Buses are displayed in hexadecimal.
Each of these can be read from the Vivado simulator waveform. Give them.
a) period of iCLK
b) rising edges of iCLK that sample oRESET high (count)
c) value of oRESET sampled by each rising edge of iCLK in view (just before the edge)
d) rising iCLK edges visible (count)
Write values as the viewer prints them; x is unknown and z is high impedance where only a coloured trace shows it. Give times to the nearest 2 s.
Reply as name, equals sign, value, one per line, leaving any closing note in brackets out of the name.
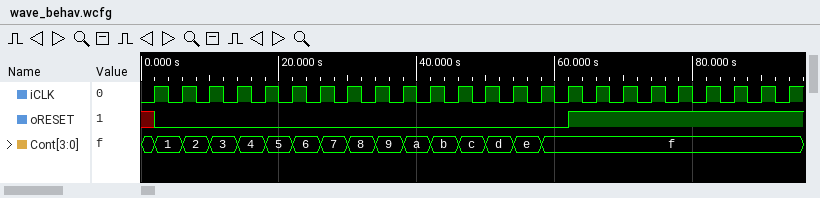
period of iCLK = 4 s
rising edges of iCLK that sample oRESET high = 8
value of oRESET sampled by each rising edge of iCLK in view = x 0 0 0 0 0 0 0 0 0 0 0 0 0 0 0 1 1 1 1 1 1 1 1
rising iCLK edges visible = 24
